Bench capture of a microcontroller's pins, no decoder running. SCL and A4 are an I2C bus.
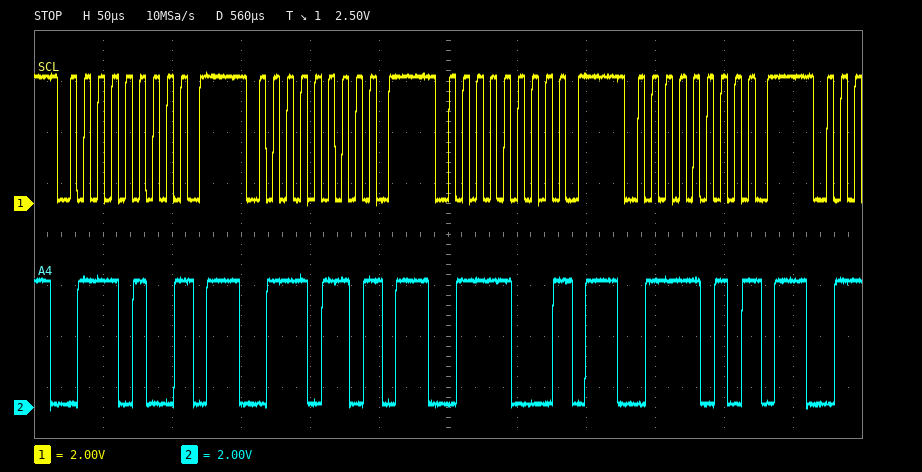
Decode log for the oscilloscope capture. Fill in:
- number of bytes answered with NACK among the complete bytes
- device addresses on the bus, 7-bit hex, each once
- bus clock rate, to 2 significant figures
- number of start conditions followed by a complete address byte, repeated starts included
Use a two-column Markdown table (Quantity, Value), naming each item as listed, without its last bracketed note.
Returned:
| Quantity | Value |
|---|---|
| number of bytes answered with NACK among the complete bytes | 4 |
| device addresses on the bus, 7-bit hex, each once | 0x3A 0x3B 0x3C 0x3D |
| bus clock rate, to 2 significant figures | 100 kHz |
| number of start conditions followed by a complete address byte, repeated starts included | 4 |
